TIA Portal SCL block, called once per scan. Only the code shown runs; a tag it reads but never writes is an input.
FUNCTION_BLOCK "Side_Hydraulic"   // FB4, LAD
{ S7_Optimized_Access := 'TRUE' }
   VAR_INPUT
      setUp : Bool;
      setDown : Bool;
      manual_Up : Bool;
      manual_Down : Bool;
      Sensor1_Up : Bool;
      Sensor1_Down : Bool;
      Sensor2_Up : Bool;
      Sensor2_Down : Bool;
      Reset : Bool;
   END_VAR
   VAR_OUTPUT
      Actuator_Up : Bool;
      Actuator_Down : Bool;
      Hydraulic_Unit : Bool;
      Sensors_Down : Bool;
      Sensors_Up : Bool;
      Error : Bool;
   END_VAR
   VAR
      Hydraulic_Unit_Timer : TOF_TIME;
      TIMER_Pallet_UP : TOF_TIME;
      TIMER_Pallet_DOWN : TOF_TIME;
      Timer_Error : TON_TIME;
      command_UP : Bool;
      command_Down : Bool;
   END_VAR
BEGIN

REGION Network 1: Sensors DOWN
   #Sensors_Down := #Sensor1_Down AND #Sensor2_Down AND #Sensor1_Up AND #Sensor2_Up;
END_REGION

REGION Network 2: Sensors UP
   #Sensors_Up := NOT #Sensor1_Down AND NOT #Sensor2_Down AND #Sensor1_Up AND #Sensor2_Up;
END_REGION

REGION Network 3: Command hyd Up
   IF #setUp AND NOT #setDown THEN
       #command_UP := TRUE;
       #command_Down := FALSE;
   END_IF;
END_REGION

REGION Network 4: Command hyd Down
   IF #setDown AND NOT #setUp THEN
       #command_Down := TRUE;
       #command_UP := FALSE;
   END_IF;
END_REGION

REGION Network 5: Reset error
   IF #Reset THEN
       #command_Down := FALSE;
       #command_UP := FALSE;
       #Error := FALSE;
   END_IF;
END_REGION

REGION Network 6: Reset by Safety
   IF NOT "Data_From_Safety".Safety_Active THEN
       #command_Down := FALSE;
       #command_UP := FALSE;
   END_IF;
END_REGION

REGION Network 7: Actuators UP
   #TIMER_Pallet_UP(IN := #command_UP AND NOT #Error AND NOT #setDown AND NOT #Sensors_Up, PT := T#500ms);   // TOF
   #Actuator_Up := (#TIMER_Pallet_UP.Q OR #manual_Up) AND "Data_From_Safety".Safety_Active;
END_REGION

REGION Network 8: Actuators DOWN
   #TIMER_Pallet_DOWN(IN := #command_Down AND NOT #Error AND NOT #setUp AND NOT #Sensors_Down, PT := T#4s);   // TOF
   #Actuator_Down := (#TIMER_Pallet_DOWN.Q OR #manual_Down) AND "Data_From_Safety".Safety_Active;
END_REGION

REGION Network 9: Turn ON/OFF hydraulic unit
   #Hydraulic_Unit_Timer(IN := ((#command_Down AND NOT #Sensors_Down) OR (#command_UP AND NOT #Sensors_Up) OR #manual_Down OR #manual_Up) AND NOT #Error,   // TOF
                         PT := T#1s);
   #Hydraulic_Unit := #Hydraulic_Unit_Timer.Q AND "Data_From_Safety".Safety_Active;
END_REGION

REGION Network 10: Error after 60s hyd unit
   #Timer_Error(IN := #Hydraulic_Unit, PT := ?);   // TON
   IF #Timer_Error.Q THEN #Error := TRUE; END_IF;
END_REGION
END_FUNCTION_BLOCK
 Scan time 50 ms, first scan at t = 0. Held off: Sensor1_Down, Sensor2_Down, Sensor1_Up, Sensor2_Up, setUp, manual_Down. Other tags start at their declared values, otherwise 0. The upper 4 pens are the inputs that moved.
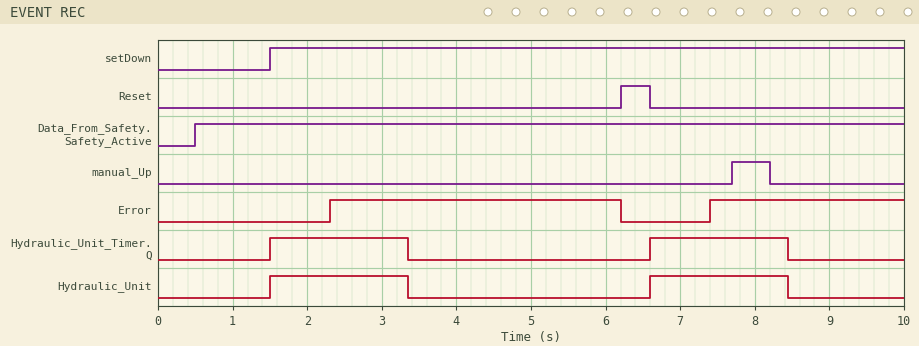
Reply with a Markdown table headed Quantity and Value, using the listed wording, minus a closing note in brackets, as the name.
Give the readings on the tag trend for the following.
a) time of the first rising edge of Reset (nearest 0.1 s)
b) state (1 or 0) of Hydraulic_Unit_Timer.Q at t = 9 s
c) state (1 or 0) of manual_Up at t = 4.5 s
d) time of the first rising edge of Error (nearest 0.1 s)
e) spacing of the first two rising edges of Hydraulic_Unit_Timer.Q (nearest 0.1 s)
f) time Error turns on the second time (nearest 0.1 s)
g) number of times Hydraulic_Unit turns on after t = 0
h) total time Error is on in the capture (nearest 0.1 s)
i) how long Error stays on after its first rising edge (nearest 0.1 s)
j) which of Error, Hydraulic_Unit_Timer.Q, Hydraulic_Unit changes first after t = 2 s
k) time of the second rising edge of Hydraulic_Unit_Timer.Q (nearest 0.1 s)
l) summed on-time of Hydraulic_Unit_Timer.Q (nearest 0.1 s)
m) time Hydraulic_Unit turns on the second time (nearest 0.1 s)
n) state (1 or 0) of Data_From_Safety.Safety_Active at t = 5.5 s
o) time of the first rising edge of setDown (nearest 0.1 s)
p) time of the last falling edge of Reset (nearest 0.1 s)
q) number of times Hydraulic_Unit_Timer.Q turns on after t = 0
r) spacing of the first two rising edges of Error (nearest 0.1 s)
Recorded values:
| Quantity | Value |
|---|---|
| time of the first rising edge of Reset | 6.2 s |
| state (1 or 0) of Hydraulic_Unit_Timer.Q at t = 9 s | 0 |
| state (1 or 0) of manual_Up at t = 4.5 s | 0 |
| time of the first rising edge of Error | 2.3 s |
| spacing of the first two rising edges of Hydraulic_Unit_Timer.Q | 5.1 s |
| time Error turns on the second time | 7.4 s |
| number of times Hydraulic_Unit turns on after t = 0 | 2 |
| total time Error is on in the capture | 6.5 s |
| how long Error stays on after its first rising edge | 3.9 s |
| which of Error, Hydraulic_Unit_Timer.Q, Hydraulic_Unit changes first after t = 2 s | Error |
| time of the second rising edge of Hydraulic_Unit_Timer.Q | 6.6 s |
| summed on-time of Hydraulic_Unit_Timer.Q | 3.7 s |
| time Hydraulic_Unit turns on the second time | 6.6 s |
| state (1 or 0) of Data_From_Safety.Safety_Active at t = 5.5 s | 1 |
| time of the first rising edge of setDown | 1.5 s |
| time of the last falling edge of Reset | 6.6 s |
| number of times Hydraulic_Unit_Timer.Q turns on after t = 0 | 2 |
| spacing of the first two rising edges of Error | 5.1 s |
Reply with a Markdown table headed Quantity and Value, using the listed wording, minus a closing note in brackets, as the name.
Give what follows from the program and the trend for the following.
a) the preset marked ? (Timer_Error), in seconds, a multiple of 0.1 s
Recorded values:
| Quantity | Value |
|---|---|
| the preset marked ? (Timer_Error), in seconds, a multiple of 0.1 s | 0.8 s |
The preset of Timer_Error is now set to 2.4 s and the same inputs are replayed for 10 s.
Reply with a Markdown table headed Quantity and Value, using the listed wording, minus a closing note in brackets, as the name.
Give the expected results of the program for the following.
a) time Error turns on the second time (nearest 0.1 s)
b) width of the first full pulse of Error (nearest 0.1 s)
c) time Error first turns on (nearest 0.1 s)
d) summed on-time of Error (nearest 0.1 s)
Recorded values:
| Quantity | Value |
|---|---|
| time Error turns on the second time | 9.0 s |
| width of the first full pulse of Error | 2.3 s |
| time Error first turns on | 3.9 s |
| summed on-time of Error | 3.3 s |
